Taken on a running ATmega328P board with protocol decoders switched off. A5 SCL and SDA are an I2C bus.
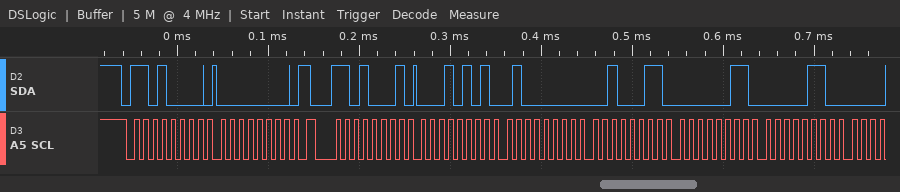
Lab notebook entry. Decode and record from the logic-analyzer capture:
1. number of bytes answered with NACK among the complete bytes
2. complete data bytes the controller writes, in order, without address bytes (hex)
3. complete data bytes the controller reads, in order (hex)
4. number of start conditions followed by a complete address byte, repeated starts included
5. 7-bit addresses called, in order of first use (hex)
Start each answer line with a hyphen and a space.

- 0
- 00
- 15 40 23 03 06
- 2
- 0x68
